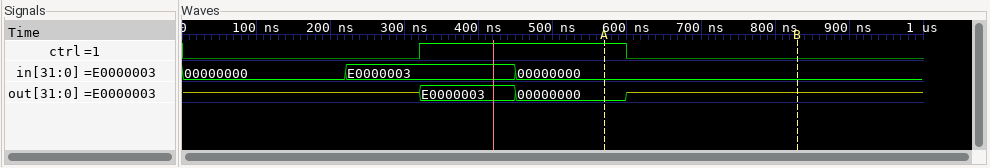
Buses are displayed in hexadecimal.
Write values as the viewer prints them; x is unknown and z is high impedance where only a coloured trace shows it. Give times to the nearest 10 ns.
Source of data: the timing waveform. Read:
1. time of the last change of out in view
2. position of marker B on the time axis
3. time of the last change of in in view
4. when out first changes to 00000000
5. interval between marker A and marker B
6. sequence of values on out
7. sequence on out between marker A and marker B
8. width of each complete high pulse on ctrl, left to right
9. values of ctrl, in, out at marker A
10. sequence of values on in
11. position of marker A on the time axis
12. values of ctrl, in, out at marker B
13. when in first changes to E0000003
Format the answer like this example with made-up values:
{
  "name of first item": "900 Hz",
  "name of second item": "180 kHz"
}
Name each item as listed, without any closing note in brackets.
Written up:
{
  "time of the last change of out in view": "600 ns",
  "position of marker B on the time axis": "830 ns",
  "time of the last change of in in view": "450 ns",
  "when out first changes to 00000000": "450 ns",
  "interval between marker A and marker B": "260 ns",
  "sequence of values on out": "z, E0000003, 00000000, z",
  "sequence on out between marker A and marker B": "00000000, z",
  "width of each complete high pulse on ctrl, left to right": "280 ns",
  "values of ctrl, in, out at marker A": "ctrl=1, in=00000000, out=00000000",
  "sequence of values on in": "00000000, E0000003, 00000000",
  "position of marker A on the time axis": "570 ns",
  "values of ctrl, in, out at marker B": "ctrl=0, in=00000000, out=z",
  "when in first changes to E0000003": "220 ns"
}
